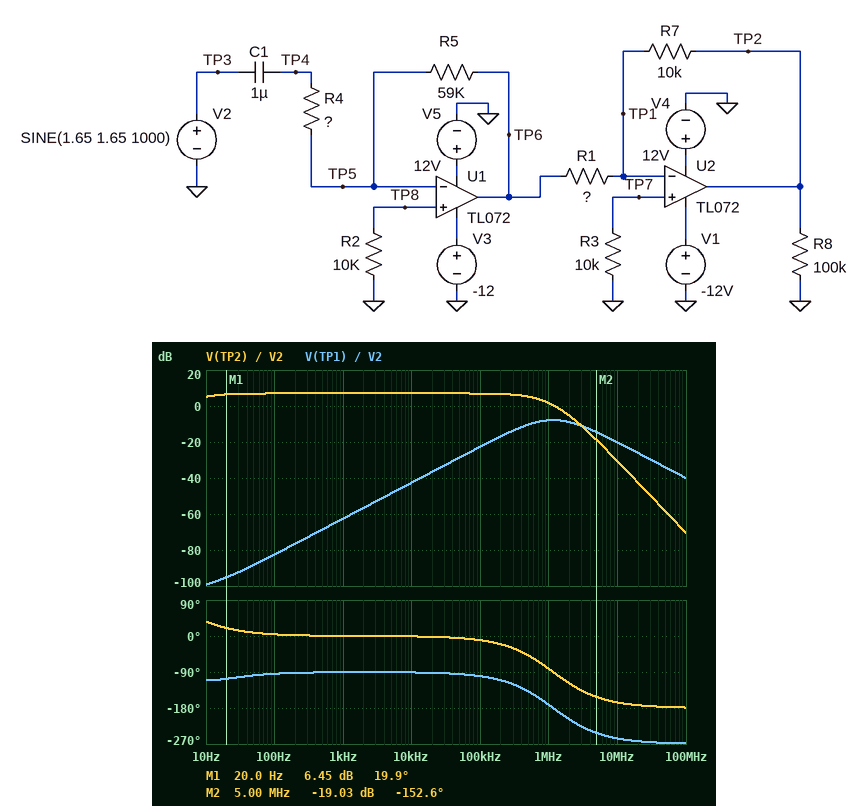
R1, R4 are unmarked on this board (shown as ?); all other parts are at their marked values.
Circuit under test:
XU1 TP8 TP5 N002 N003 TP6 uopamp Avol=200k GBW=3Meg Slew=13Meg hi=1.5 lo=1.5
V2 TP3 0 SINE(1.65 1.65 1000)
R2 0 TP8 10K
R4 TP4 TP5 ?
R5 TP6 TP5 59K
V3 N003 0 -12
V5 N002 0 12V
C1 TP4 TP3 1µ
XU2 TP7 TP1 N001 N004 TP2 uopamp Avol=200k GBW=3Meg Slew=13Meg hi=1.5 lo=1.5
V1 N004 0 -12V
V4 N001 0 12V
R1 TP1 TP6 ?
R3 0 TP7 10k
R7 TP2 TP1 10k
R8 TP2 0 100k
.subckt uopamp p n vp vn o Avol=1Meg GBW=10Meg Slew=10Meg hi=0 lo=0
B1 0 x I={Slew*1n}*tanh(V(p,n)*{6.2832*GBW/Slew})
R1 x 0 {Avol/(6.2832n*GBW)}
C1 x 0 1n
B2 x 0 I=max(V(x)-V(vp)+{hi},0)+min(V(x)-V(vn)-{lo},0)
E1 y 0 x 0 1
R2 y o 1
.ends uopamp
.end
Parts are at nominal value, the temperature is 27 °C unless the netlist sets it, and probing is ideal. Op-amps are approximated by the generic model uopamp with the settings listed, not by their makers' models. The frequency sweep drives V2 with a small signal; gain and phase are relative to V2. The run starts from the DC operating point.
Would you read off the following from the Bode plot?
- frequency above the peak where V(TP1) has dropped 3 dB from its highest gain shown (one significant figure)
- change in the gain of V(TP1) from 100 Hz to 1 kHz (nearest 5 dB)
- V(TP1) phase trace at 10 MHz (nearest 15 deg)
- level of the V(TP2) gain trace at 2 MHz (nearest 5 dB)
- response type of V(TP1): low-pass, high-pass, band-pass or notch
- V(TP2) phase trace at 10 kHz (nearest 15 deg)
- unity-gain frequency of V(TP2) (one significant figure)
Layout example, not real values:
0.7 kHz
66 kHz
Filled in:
3 MHz
20 dB
-255 deg
-5 dB
band-pass
0 deg
1 MHz
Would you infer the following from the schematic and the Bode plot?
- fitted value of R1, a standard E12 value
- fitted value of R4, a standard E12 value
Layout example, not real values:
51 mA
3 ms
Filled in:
12 kΩ
22 kΩ
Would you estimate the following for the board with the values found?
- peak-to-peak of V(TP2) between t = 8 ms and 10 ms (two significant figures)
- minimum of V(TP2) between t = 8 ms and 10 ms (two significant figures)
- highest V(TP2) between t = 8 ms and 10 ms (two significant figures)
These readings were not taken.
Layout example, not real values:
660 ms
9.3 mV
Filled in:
7.4 V
-3.7 V
3.7 V
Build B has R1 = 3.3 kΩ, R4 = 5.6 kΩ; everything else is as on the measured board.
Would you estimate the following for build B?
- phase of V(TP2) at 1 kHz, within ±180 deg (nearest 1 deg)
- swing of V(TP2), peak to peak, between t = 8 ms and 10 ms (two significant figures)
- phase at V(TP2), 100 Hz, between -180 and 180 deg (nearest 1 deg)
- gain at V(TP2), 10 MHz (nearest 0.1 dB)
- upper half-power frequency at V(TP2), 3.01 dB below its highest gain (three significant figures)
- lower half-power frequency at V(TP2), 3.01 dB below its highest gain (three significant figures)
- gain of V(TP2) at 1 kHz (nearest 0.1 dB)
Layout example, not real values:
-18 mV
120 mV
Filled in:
1 deg
21 V
16 deg
-24.2 dB
235 kHz
28.4 Hz
30.1 dB
